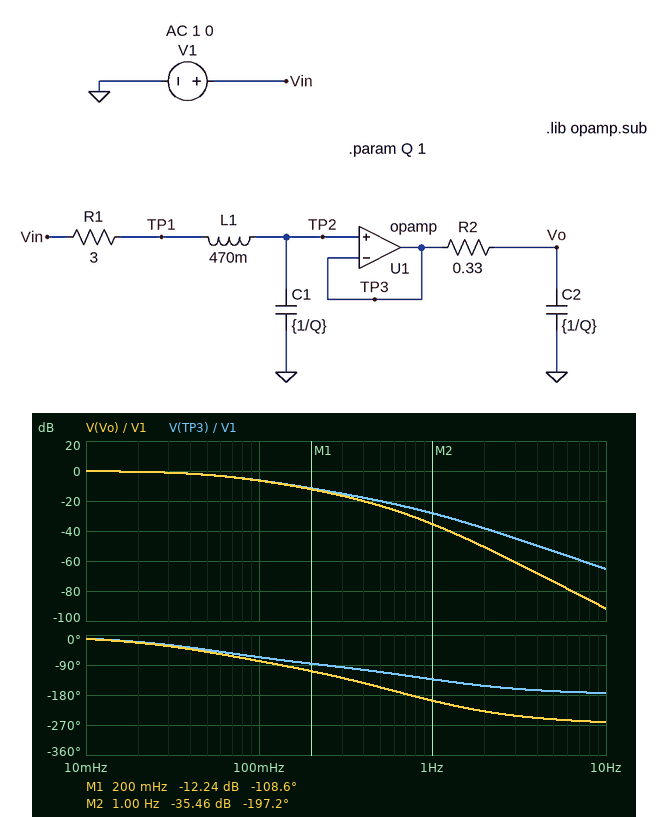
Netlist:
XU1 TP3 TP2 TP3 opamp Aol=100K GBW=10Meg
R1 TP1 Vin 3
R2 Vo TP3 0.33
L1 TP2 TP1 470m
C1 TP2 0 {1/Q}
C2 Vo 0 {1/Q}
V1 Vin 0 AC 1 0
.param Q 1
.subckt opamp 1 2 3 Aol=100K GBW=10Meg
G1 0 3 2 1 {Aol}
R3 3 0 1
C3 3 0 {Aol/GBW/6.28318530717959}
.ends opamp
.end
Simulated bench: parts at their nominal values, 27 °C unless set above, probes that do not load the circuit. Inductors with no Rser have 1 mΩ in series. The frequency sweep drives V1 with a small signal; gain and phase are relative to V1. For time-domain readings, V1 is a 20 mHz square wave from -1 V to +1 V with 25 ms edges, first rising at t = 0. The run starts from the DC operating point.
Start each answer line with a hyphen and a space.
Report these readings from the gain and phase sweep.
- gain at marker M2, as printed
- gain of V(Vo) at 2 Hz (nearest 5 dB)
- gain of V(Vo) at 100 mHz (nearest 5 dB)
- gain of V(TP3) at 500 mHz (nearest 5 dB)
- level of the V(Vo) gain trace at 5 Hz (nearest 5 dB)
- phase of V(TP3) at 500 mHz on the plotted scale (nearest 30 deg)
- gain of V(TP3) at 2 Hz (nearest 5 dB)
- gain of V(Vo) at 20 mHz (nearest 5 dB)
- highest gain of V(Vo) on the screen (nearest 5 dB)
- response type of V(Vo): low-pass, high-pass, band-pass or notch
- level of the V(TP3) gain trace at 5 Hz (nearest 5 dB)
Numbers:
- -35.46 dB
- -50 dB
- -5 dB
- -20 dB
- -75 dB
- -120 deg
- -40 dB
- 0 dB
- 0 dB
- low-pass
- -55 dB
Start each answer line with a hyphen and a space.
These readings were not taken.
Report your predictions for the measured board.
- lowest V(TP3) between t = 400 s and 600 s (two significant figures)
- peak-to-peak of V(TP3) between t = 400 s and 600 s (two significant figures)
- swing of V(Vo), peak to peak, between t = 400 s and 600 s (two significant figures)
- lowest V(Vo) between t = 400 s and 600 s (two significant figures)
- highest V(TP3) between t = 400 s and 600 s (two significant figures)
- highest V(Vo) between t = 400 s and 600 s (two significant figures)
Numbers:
- -1.0 V
- 2.0 V
- 2.0 V
- -1.0 V
- 1.0 V
- 1.0 V
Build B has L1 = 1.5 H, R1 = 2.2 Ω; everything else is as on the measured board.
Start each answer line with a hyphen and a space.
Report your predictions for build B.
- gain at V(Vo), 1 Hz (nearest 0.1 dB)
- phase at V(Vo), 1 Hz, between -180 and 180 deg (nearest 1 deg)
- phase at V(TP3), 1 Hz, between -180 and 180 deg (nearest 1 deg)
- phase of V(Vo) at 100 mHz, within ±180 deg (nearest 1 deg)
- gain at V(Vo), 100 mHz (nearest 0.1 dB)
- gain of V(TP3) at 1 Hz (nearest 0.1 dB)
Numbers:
- -42.8 dB
- 129 deg
- -167 deg
- -85 deg
- -3.4 dB
- -35.5 dB
